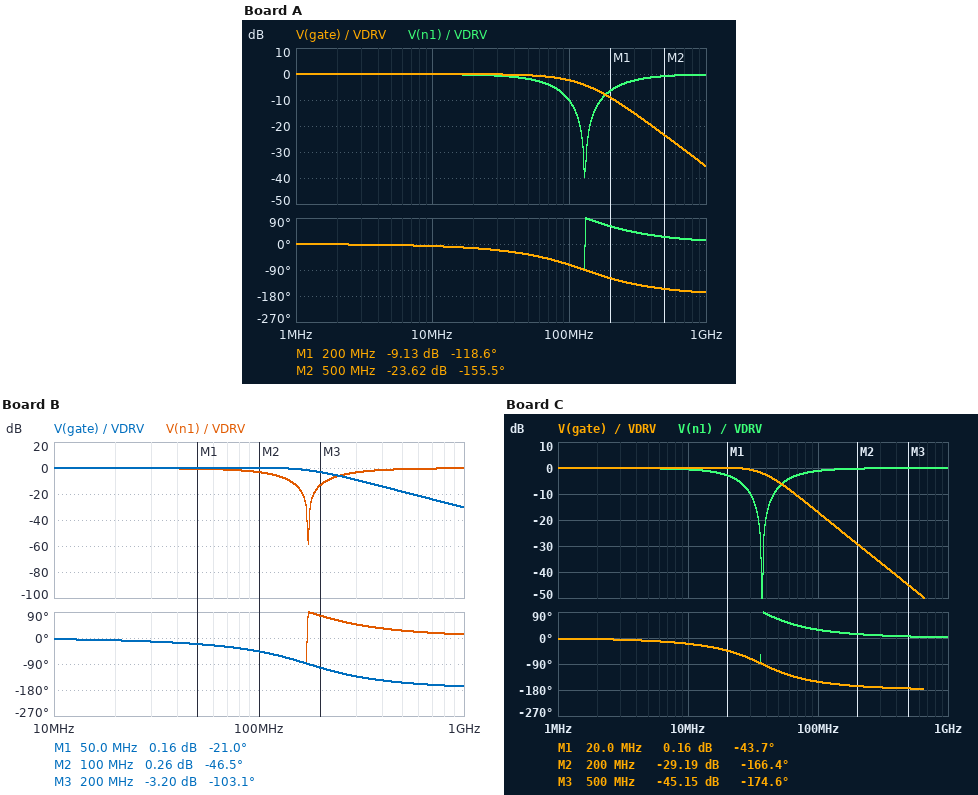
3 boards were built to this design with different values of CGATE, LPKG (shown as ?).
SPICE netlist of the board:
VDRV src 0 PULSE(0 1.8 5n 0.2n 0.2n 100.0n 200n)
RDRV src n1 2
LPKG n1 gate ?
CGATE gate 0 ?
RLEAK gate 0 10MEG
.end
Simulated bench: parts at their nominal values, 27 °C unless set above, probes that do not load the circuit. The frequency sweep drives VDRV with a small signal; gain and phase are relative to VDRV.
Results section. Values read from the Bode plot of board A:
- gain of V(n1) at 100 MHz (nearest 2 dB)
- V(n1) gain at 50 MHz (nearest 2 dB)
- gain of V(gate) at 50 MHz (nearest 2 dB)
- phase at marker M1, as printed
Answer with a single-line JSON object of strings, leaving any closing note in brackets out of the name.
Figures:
{"gain of V(n1) at 100 MHz": "-10 dB", "V(n1) gain at 50 MHz": "-2 dB", "gain of V(gate) at 50 MHz": "0 dB", "phase at marker M1, as printed": "-118.6 deg"}
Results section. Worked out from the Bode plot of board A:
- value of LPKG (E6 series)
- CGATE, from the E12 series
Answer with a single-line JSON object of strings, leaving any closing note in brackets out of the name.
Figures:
{"value of LPKG": "1.5 nH", "CGATE, from the E12 series": "1 nF"}
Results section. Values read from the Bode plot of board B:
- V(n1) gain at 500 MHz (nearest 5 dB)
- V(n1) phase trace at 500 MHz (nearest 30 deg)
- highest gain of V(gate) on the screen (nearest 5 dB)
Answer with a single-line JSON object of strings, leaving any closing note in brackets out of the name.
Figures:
{"V(n1) gain at 500 MHz": "0 dB", "V(n1) phase trace at 500 MHz": "30 deg", "highest gain of V(gate) on the screen": "0 dB"}
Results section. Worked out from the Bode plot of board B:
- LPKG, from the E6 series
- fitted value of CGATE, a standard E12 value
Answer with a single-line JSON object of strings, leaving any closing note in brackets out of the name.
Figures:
{"LPKG, from the E6 series": "1.5 nH", "fitted value of CGATE, a standard E12 value": "560 pF"}
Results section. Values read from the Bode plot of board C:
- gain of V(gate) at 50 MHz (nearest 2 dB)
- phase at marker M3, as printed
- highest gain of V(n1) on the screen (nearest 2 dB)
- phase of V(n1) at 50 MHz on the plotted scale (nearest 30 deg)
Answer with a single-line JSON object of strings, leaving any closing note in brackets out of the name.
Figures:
{"gain of V(gate) at 50 MHz": "-6 dB", "phase at marker M3, as printed": "-174.6 deg", "highest gain of V(n1) on the screen": "0 dB", "phase of V(n1) at 50 MHz on the plotted scale": "60 deg"}
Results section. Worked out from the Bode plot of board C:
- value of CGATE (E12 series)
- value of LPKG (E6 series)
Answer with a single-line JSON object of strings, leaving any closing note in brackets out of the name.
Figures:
{"value of CGATE": "2.7 nF", "value of LPKG": "6.8 nH"}
